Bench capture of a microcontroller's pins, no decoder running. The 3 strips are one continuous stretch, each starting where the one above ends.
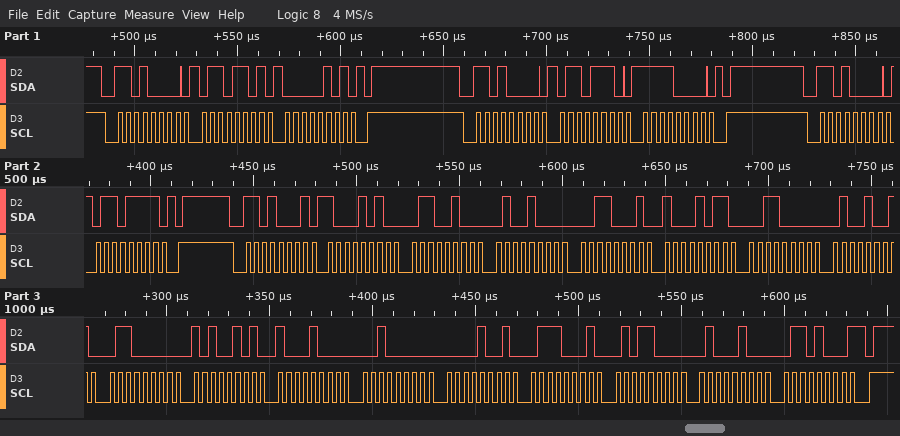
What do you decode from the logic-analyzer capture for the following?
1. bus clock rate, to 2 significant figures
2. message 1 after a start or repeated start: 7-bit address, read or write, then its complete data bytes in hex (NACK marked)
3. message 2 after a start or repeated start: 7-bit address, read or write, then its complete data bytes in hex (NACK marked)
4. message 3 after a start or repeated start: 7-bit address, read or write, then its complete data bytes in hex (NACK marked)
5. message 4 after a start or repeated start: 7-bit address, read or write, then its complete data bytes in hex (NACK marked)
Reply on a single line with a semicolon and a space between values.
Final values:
250 kHz; 0x68 write: 6D 05; 0x68 write: 6E F0; 0x68 write: 6F; 0x68 read: 8A 64 48 31 8B 30 49 60 A5 88 20 09 71 58 44 68 NACK
